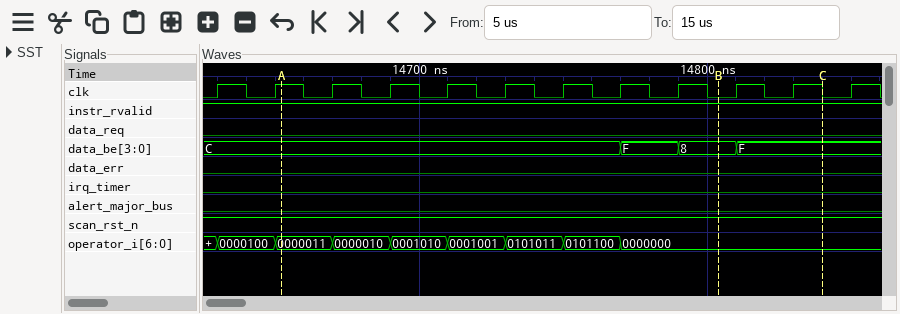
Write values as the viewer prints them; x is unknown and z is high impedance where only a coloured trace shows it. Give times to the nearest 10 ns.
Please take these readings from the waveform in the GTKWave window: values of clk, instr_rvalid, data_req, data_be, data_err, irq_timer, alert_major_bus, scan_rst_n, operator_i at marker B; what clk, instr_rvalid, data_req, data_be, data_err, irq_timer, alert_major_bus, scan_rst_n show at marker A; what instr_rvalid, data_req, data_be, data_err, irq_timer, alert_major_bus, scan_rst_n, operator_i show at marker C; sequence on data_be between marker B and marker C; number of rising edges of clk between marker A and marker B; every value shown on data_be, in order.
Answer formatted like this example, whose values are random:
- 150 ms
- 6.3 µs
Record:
- clk=0, instr_rvalid=1, data_req=0, data_be=8, data_err=0, irq_timer=0, alert_major_bus=0, scan_rst_n=1, operator_i=0000000
- clk=1, instr_rvalid=1, data_req=0, data_be=C, data_err=0, irq_timer=0, alert_major_bus=0, scan_rst_n=1
- instr_rvalid=1, data_req=0, data_be=F, data_err=0, irq_timer=0, alert_major_bus=0, scan_rst_n=1, operator_i=0000000
- 8, F
- 7
- C, F, 8, F
